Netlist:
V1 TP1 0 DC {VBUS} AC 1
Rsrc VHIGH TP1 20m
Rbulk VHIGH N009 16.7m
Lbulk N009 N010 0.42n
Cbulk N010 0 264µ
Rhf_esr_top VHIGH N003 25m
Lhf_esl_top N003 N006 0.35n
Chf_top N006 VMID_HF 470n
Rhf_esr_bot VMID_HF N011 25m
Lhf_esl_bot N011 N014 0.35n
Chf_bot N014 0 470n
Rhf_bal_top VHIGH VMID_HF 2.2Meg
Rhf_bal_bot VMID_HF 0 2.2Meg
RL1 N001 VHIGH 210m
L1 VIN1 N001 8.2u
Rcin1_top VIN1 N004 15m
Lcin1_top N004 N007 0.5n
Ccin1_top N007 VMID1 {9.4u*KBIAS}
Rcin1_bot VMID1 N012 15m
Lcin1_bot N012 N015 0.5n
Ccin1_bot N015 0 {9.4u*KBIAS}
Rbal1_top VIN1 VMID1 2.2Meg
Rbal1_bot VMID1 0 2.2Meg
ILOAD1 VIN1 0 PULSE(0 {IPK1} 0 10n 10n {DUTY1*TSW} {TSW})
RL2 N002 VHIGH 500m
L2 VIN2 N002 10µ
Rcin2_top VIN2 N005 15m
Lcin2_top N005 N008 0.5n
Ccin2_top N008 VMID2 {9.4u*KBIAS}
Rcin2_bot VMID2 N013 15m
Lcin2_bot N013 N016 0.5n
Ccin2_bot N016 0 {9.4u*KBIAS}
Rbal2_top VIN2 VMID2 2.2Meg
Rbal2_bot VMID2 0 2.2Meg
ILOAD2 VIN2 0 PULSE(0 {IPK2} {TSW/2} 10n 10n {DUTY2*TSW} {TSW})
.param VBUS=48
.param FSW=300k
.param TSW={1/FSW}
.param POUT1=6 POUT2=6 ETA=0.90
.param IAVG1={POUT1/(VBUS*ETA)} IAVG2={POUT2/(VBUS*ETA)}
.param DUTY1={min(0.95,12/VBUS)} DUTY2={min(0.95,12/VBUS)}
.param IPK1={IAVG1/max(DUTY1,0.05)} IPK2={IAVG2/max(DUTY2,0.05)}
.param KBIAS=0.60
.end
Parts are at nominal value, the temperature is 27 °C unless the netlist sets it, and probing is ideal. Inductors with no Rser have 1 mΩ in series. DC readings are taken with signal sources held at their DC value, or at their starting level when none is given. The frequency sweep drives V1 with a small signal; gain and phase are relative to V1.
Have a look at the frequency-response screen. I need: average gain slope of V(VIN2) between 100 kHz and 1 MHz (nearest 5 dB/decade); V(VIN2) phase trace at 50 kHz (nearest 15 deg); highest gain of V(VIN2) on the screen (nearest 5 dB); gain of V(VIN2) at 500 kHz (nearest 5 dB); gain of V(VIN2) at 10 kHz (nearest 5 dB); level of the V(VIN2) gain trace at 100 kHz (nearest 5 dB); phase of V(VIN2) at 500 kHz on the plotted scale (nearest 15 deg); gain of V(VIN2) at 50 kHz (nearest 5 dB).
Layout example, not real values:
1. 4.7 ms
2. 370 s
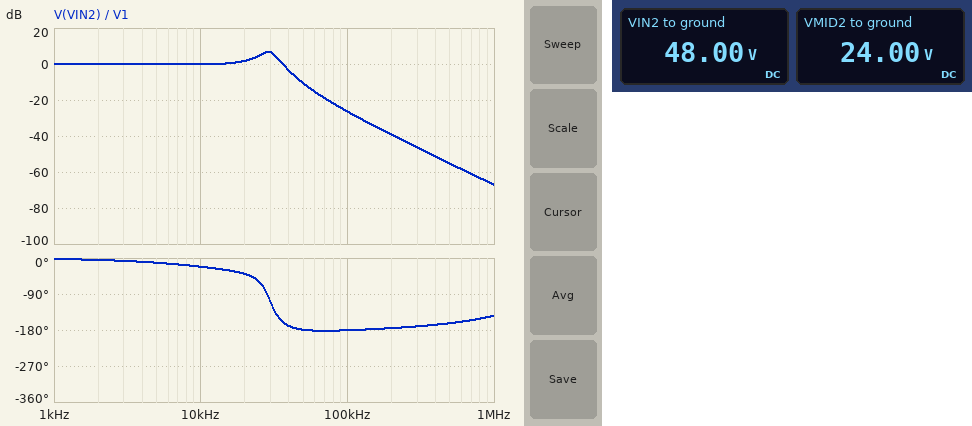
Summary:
1. -40 dB/decade
2. -180 deg
3. 5 dB
4. -55 dB
5. 0 dB
6. -25 dB
7. -165 deg
8. -10 dB
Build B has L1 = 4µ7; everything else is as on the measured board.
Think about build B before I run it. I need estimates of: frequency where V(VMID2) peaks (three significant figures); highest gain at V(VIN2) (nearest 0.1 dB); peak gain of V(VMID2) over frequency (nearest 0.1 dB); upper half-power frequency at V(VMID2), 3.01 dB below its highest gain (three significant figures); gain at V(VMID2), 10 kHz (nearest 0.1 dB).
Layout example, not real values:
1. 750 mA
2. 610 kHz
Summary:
1. 29.1 kHz
2. 6.8 dB
3. 0.8 dB
4. 33.1 kHz
5. -6.1 dB
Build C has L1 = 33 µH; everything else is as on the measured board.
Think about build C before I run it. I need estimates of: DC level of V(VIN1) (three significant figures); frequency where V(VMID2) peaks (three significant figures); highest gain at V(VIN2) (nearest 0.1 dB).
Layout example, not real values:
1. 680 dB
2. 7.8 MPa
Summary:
1. 48.0 V
2. 29.1 kHz
3. 6.9 dB
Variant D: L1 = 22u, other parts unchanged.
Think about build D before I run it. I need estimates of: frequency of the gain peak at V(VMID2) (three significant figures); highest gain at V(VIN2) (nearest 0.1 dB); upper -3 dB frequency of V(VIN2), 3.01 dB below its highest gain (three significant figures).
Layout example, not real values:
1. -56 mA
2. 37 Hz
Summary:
1. 29.1 kHz
2. 6.9 dB
3. 33.1 kHz
